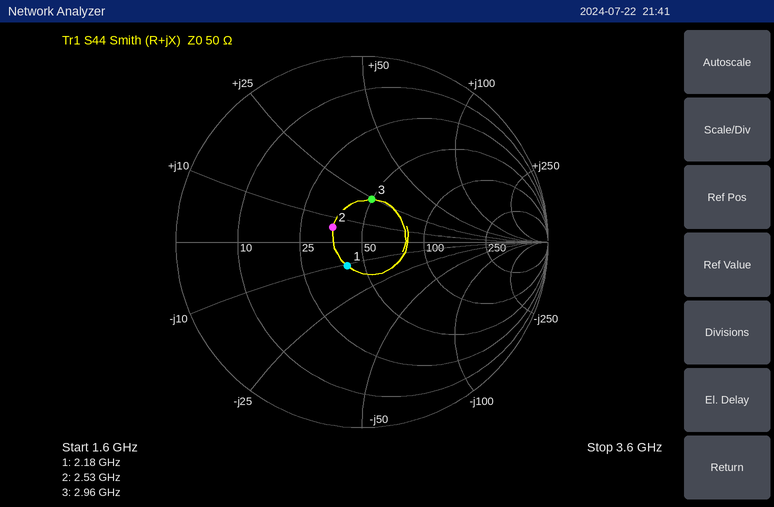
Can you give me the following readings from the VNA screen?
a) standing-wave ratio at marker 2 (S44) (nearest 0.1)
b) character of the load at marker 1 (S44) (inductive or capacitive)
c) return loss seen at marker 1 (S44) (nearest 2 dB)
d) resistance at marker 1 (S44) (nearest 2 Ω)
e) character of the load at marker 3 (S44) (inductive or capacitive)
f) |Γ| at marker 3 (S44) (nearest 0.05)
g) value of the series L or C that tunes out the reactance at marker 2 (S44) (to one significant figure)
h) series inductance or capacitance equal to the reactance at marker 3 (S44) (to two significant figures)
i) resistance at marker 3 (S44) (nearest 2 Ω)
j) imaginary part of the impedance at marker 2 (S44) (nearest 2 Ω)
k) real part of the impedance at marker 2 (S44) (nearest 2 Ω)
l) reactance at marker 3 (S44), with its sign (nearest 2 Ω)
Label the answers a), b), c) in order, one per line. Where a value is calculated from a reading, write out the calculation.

a) 1.4
b) capacitive
c) 16 dB
d) 42 Ω
e) inductive
f) 0.25
g) C = 1/(2π × 2.53 GHz × 6 Ω) ≈ 10 pF
h) L = 24 Ω/(2π × 2.96 GHz) ≈ 1.3 nH
i) 50 Ω
j) +6 Ω
k) 36 Ω
l) +24 Ω
